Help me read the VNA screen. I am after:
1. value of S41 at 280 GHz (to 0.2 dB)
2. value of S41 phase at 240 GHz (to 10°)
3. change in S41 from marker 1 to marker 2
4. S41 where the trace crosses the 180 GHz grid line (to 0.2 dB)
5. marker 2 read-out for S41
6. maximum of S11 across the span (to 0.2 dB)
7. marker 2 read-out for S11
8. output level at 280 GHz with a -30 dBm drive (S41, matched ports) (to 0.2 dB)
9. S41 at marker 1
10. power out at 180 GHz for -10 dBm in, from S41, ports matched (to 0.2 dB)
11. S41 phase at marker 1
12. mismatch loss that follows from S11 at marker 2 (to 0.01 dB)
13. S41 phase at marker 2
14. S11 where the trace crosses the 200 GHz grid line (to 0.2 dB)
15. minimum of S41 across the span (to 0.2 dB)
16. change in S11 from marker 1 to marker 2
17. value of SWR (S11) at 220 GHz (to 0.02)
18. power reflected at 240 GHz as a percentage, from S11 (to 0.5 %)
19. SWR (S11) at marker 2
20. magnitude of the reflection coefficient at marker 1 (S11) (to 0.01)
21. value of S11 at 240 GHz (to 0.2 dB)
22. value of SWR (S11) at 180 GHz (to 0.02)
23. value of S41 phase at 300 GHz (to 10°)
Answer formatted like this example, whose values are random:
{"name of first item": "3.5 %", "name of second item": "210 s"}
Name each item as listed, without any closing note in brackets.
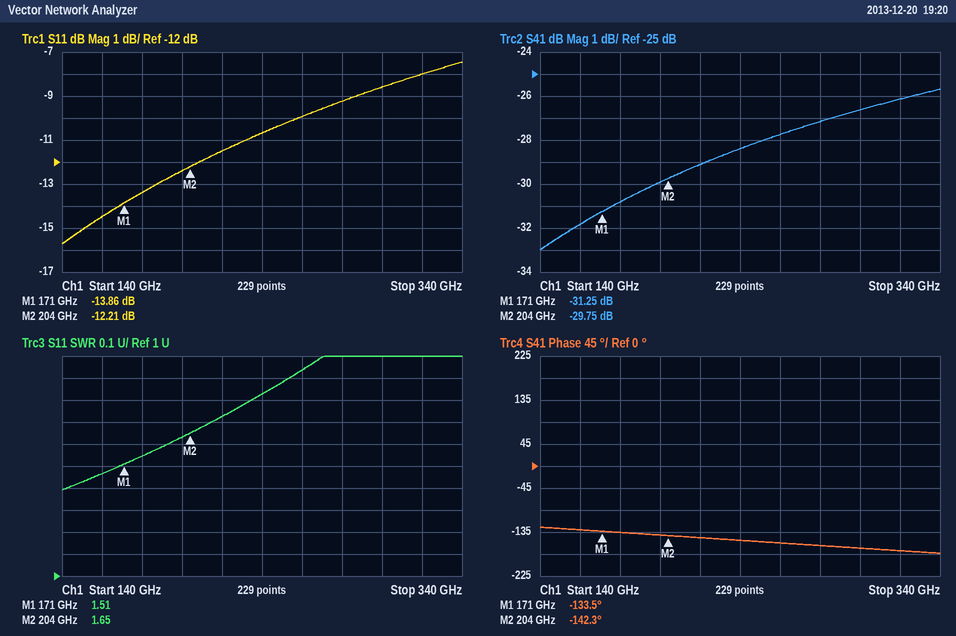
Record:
{"value of S41 at 280 GHz": "-27.2 dB", "value of S41 phase at 240 GHz": "-150°", "change in S41 from marker 1 to marker 2": "1.50 dB", "S41 where the trace crosses the 180 GHz grid line": "-30.8 dB", "marker 2 read-out for S41": "-29.75 dB", "maximum of S11 across the span": "-7.4 dB", "marker 2 read-out for S11": "-12.21 dB", "output level at 280 GHz with a -30 dBm drive (S41, matched ports)": "-57.2 dBm", "S41 at marker 1": "-31.25 dB", "power out at 180 GHz for -10 dBm in, from S41, ports matched": "-40.8 dBm", "S41 phase at marker 1": "-133.5°", "mismatch loss that follows from S11 at marker 2": "0.27 dB", "S41 phase at marker 2": "-142.3°", "S11 where the trace crosses the 200 GHz grid line": "-12.4 dB", "minimum of S41 across the span": "-33.0 dB", "change in S11 from marker 1 to marker 2": "1.65 dB", "value of SWR (S11) at 220 GHz": "1.72", "power reflected at 240 GHz as a percentage, from S11": "8.5 %", "SWR (S11) at marker 2": "1.65", "magnitude of the reflection coefficient at marker 1 (S11)": "0.20", "value of S11 at 240 GHz": "-10.6 dB", "value of SWR (S11) at 180 GHz": "1.54", "value of S41 phase at 300 GHz": "-170°"}
